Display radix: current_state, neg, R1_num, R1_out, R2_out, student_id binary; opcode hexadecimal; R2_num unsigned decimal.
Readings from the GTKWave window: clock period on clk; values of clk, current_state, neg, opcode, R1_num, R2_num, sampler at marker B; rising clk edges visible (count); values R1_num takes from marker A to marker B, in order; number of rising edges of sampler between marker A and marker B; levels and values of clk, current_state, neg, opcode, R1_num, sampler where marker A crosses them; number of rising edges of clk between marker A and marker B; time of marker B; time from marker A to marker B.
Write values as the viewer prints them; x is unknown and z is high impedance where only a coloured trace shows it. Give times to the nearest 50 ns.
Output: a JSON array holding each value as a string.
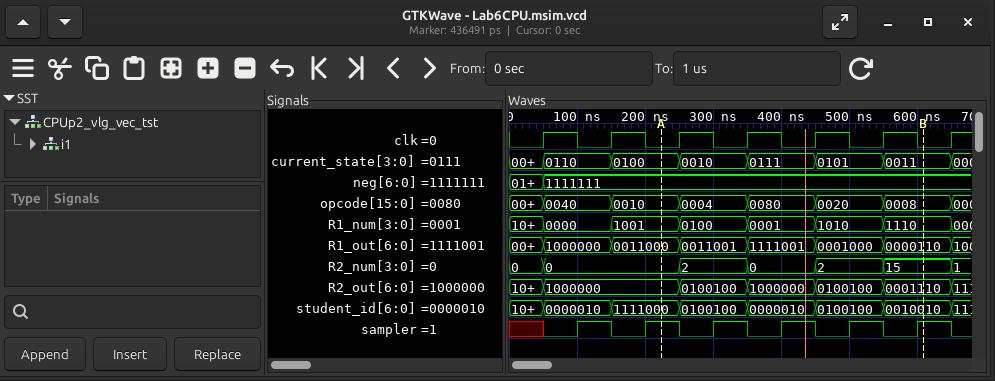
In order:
["100 ns", "clk=0, current_state=0011, neg=1111111, opcode=0008, R1_num=1110, R2_num=15, sampler=1", "7", "1001, 0100, 0001, 1010, 1110", "4", "clk=0, current_state=0100, neg=1111111, opcode=0010, R1_num=1001, sampler=1", "4", "600 ns", "400 ns"]
